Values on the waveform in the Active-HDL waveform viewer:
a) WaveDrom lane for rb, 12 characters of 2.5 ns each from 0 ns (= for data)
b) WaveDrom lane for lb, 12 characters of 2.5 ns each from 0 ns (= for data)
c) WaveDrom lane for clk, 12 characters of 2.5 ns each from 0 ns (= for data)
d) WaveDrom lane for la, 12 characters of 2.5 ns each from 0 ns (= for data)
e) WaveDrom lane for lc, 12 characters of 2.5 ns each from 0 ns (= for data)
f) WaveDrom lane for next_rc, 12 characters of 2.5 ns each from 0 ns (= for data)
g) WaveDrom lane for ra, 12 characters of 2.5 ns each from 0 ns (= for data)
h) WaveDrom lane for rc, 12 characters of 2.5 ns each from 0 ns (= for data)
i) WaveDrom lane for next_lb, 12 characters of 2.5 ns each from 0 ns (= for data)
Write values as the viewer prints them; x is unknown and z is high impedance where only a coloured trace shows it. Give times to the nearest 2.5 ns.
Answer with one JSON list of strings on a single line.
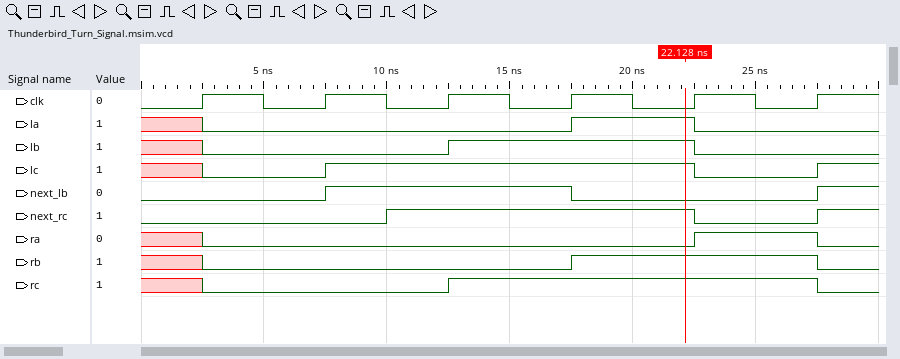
["{name: 'rb', wave: 'x0.....1...0'}", "{name: 'lb', wave: 'x0...1...0..'}", "{name: 'clk', wave: '010101010101'}", "{name: 'la', wave: 'x0.....1.0..'}", "{name: 'lc', wave: 'x0.1.....0.1'}", "{name: 'next_rc', wave: '0...1....0.1'}", "{name: 'ra', wave: 'x0.......1.0'}", "{name: 'rc', wave: 'x0...1.....0'}", "{name: 'next_lb', wave: '0..1...0...1'}"]
